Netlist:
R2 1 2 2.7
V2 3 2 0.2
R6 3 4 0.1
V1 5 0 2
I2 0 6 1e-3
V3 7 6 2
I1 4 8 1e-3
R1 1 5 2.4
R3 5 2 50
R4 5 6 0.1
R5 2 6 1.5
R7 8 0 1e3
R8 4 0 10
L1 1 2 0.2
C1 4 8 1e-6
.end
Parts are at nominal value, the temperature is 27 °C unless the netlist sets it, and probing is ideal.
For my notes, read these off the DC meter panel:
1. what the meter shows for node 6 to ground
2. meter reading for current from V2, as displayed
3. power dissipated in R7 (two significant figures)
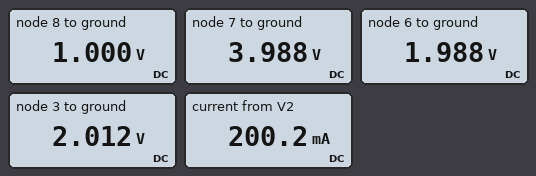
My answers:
1.988 V
200.2 mA
1.0 mW
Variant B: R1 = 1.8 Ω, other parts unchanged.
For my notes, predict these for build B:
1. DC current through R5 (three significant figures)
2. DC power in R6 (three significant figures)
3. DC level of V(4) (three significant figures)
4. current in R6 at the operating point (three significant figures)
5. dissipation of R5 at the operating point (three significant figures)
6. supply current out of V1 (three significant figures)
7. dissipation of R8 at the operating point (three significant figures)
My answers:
105 mA
4.09 mW
2.01 V
202 mA
16.6 mW
201 mA
405 mW
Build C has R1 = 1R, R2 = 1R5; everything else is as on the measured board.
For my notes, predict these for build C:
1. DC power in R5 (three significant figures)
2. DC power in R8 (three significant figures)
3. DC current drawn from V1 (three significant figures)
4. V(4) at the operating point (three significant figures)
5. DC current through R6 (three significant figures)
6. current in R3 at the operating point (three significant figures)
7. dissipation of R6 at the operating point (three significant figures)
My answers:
9.23 mW
422 mW
205 mA
2.05 V
206 mA
2.51 mA
4.26 mW
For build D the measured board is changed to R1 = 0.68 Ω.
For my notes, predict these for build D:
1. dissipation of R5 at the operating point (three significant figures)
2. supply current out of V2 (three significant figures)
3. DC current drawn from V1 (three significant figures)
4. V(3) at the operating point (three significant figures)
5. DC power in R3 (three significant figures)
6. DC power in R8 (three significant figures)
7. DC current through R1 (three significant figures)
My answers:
5.73 mW
209 mA
208 mA
2.10 V
195 µW
433 mW
145 mA
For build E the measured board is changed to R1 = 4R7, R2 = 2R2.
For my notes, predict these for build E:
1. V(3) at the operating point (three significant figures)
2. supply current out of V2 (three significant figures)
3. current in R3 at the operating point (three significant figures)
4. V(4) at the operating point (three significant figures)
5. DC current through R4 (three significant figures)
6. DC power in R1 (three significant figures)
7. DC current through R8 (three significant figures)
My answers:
1.97 V
196 mA
4.57 mA
1.95 V
142 mA
11.1 mW
195 mA
